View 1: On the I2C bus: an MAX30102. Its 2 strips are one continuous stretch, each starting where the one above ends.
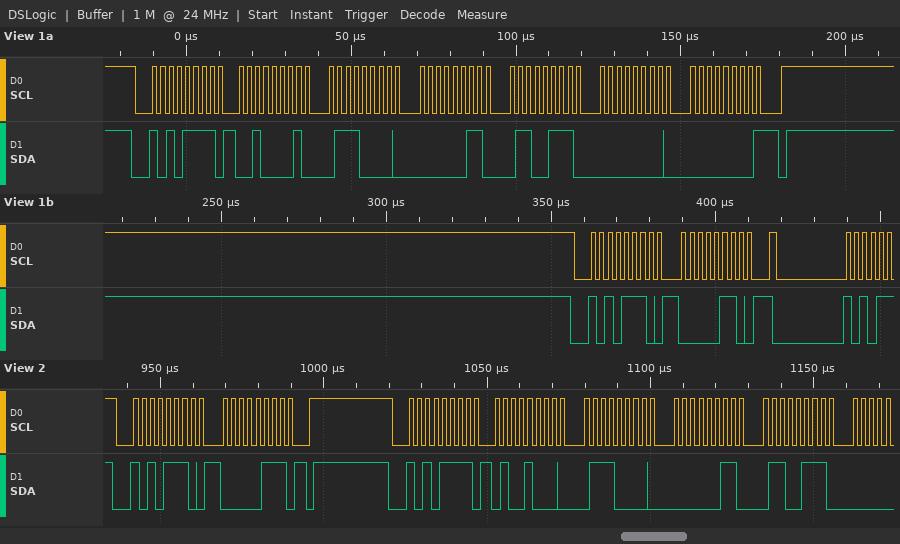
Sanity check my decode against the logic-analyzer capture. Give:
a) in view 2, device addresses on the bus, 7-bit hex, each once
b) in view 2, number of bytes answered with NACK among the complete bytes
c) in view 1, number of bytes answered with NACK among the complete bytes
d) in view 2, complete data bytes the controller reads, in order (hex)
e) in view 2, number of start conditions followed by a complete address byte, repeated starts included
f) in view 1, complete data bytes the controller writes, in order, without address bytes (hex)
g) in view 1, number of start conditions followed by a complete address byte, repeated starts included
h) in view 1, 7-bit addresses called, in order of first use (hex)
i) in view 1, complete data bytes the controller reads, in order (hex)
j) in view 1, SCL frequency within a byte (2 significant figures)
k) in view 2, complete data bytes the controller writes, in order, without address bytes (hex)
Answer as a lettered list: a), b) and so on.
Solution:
a) 0x57
b) 0
c) 1
d) 48 70 03 67
e) 2
f) 06
g) 2
h) 0x57
i) 21 70 03 67 00 00
j) 400 kHz
k) 07
